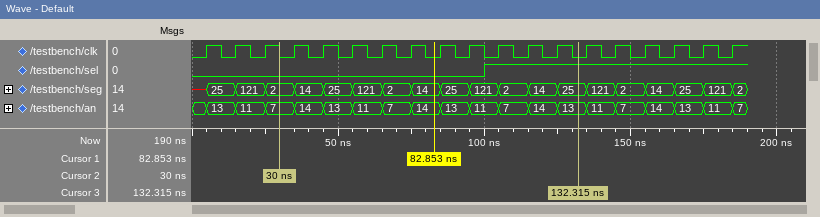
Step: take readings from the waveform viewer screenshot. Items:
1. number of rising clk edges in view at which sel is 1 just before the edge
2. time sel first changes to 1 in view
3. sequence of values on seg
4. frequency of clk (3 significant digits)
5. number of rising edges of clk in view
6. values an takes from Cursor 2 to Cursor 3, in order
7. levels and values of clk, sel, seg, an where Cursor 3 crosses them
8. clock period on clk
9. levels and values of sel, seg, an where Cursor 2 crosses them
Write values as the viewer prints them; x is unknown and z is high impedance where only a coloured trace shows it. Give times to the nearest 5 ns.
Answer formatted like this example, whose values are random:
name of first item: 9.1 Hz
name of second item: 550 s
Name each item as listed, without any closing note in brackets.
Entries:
number of rising clk edges in view at which sel is 1 just before the edge: 9
time sel first changes to 1 in view: 100 ns
sequence of values on seg: x, 25, 121, 2, 14, 25, 121, 2, 14, 25, 121, 2, 14, 25, 121, 2, 14, 25, 121, 2
frequency of clk: 100 MHz
number of rising edges of clk in view: 19
values an takes from Cursor 2 to Cursor 3, in order: 7, 14, 13, 11, 7, 14, 13, 11, 7, 14, 13
levels and values of clk, sel, seg, an where Cursor 3 crosses them: clk=0, sel=1, seg=25, an=13
clock period on clk: 10 ns
levels and values of sel, seg, an where Cursor 2 crosses them: sel=0, seg=2, an=7
